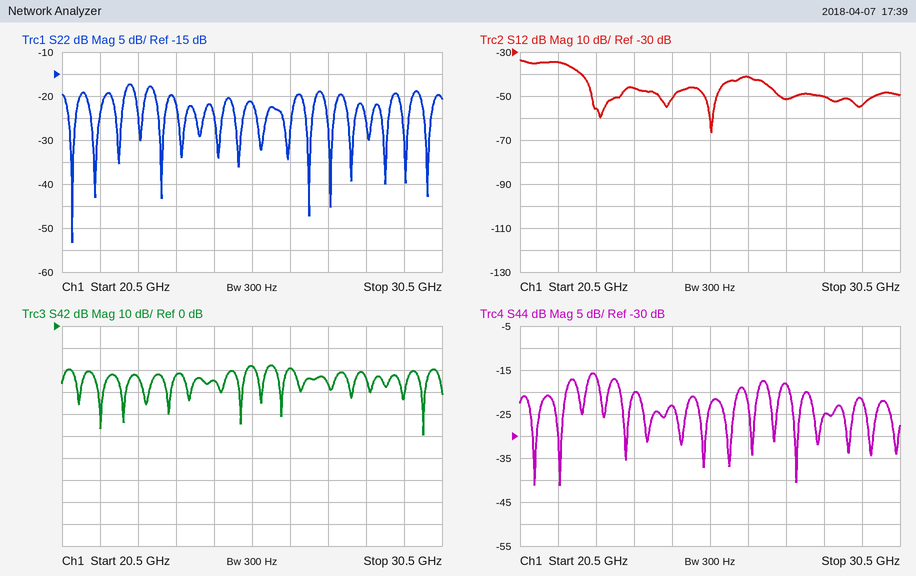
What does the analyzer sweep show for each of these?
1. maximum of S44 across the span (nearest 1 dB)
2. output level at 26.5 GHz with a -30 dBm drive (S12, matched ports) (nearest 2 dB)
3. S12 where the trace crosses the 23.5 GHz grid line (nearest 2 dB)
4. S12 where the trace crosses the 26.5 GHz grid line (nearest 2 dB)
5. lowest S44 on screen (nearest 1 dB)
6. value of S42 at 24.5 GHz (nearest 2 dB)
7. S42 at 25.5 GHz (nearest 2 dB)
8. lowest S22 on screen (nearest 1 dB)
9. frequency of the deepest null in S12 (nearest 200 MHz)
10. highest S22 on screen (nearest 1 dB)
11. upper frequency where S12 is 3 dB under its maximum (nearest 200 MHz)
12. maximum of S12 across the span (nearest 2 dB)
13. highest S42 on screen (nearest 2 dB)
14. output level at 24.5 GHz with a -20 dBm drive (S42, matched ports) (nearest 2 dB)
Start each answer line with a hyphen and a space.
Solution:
- -16 dB
- -72 dBm
- -46 dB
- -42 dB
- -41 dB
- -24 dB
- -18 dB
- -53 dB
- 25.6 GHz
- -17 dB
- 21.8 GHz
- -34 dB
- -18 dB
- -44 dBm
